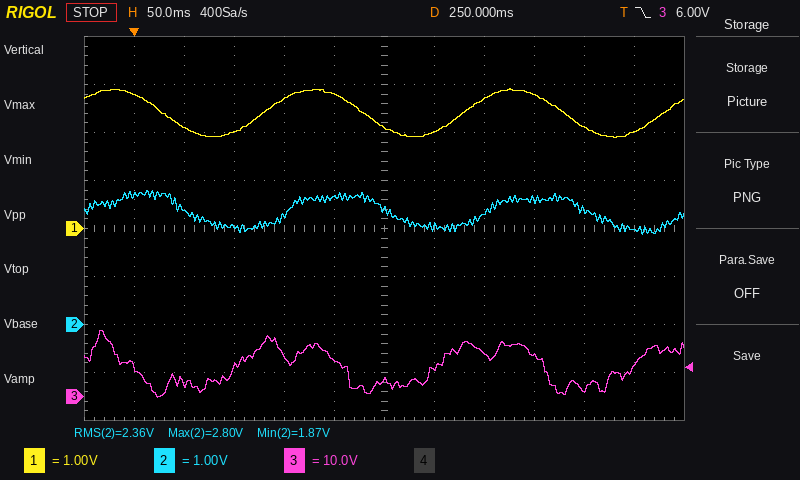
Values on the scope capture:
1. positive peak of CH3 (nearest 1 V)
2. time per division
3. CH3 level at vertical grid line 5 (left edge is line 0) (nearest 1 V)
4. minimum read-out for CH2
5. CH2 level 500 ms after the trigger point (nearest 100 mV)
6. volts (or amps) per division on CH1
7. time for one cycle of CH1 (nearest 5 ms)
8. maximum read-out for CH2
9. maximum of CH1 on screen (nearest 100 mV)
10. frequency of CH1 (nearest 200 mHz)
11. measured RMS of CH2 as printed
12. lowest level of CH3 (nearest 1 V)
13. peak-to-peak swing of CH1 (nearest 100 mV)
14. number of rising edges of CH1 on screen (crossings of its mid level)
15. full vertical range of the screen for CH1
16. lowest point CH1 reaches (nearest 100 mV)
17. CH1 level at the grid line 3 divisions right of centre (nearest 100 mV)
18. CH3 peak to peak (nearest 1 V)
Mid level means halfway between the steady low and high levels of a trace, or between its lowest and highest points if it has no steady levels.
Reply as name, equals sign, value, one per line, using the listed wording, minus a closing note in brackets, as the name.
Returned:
positive peak of CH3 = 14 V
time per division = 50 ms
CH3 level at vertical grid line 5 (left edge is line 0) = 8 V
minimum read-out for CH2 = 1.87 V
CH2 level 500 ms after the trigger point = 2.0 V
volts (or amps) per division on CH1 = 1 V
time for one cycle of CH1 = 200 ms
maximum read-out for CH2 = 2.80 V
maximum of CH1 on screen = 2.9 V
frequency of CH1 = 5.0 Hz
measured RMS of CH2 as printed = 2.36 V
lowest level of CH3 = 0 V
peak-to-peak swing of CH1 = 1.0 V
number of rising edges of CH1 on screen = 3
full vertical range of the screen for CH1 = 8 V
lowest point CH1 reaches = 1.9 V
CH1 level at the grid line 3 divisions right of centre = 2.8 V
CH3 peak to peak = 14 V
